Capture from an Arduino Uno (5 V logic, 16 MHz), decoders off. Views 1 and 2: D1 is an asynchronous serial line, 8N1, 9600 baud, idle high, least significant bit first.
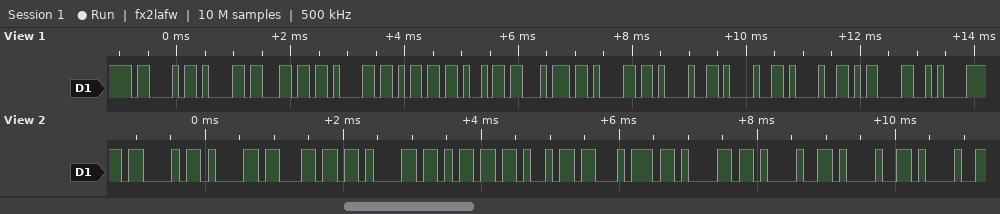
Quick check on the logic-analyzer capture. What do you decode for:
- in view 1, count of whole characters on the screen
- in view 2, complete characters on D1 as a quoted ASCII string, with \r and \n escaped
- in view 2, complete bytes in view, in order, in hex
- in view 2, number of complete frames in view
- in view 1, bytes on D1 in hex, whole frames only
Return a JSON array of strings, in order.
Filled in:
["13", "\"Calamita!!!\"", "43 61 6C 61 6D 69 74 61 21 21 21", "11", "43 61 6C 61 6D 69 74 61 21 21 21 0D 0A"]
